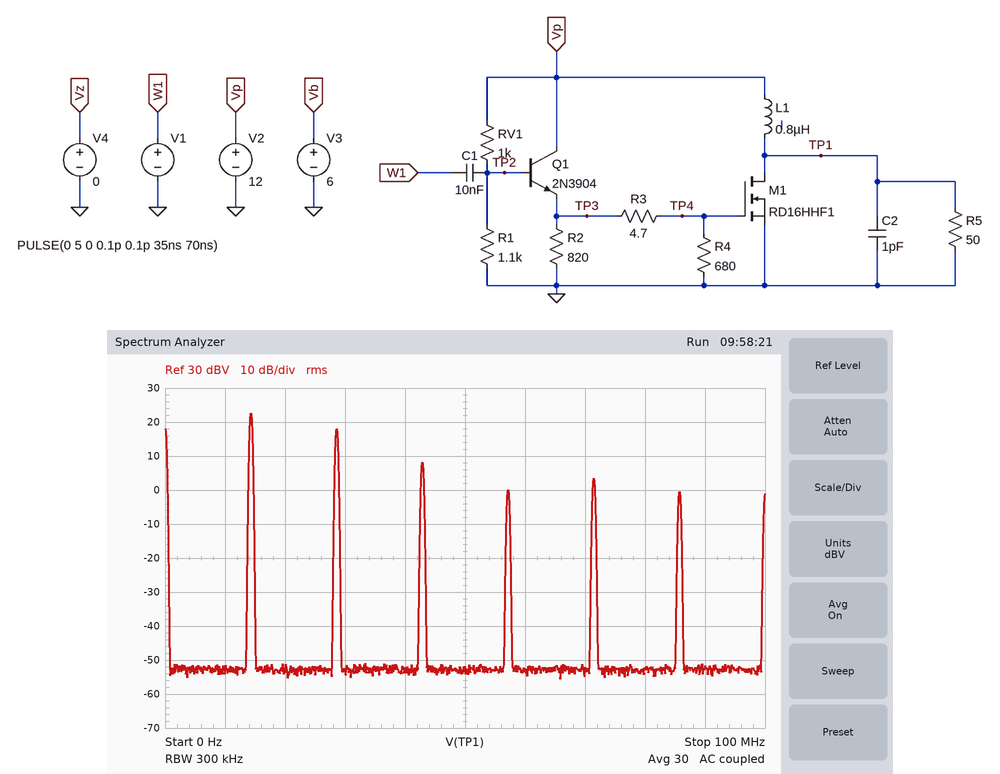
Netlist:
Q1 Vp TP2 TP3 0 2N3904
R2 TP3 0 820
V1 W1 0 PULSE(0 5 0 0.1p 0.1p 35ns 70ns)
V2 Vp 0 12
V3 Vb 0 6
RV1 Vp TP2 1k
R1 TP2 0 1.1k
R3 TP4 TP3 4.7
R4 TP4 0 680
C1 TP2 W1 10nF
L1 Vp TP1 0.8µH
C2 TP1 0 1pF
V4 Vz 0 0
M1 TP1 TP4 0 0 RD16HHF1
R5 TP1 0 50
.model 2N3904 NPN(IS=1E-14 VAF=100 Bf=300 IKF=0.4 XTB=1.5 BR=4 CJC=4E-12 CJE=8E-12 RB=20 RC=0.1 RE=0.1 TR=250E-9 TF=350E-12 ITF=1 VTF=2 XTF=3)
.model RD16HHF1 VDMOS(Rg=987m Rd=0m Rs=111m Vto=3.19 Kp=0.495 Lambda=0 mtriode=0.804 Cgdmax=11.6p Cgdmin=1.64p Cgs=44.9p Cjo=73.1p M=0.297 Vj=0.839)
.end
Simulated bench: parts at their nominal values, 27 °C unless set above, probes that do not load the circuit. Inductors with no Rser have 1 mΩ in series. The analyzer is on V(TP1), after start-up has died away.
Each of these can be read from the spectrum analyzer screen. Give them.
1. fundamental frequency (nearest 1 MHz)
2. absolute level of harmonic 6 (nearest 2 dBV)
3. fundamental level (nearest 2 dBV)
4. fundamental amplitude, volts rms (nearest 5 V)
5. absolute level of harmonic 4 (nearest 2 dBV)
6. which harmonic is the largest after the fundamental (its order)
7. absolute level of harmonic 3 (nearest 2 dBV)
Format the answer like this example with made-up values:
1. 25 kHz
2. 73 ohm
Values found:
1. 14 MHz
2. 0 dBV
3. 22 dBV
4. 15 V
5. 0 dBV
6. 2
7. 8 dBV
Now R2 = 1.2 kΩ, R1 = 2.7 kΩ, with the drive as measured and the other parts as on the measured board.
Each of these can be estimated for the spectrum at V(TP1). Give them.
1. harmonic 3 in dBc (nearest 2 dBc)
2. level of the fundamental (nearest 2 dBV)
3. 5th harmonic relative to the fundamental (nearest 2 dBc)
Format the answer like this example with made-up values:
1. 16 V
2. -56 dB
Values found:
1. -8 dBc
2. 22 dBV
3. -22 dBc
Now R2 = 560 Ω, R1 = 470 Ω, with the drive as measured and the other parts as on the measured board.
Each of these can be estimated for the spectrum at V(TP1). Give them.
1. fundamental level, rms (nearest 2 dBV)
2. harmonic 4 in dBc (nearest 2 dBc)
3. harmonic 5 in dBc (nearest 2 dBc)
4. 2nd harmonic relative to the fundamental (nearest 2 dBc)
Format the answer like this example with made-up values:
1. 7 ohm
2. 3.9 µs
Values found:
1. 22 dBV
2. -16 dBc
3. -30 dBc
4. -10 dBc
